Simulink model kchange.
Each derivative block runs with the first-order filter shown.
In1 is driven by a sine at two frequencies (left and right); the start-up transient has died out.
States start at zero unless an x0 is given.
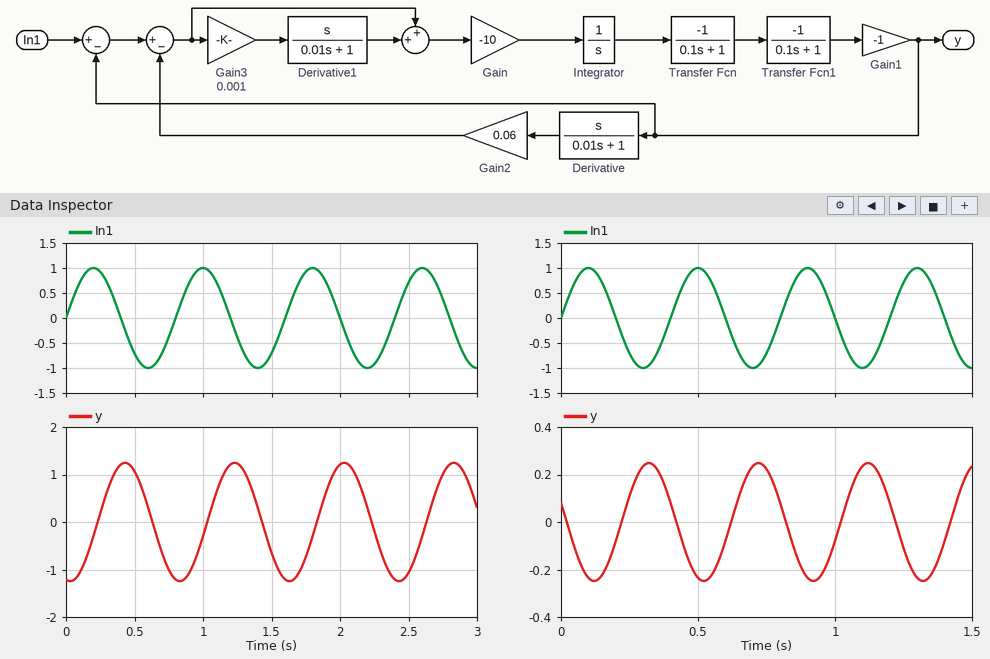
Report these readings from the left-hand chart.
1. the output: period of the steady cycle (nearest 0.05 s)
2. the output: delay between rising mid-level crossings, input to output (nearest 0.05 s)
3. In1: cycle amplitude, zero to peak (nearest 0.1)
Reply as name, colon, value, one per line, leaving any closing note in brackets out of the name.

the output: period of the steady cycle: 0.80 s
the output: delay between rising mid-level crossings, input to output: 0.25 s
In1: cycle amplitude, zero to peak: 1.0
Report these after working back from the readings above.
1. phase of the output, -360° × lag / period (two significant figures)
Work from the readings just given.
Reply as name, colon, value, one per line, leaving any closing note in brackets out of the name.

phase of the output, -360° × lag / period: -110°
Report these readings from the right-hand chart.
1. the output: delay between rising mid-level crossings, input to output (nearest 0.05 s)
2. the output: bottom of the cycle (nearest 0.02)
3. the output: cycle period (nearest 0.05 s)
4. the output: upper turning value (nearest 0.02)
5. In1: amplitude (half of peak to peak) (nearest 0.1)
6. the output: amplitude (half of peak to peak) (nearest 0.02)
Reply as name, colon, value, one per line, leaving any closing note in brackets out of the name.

the output: delay between rising mid-level crossings, input to output: 0.20 s
the output: bottom of the cycle: -0.24
the output: cycle period: 0.40 s
the output: upper turning value: 0.24
In1: amplitude (half of peak to peak): 1.0
the output: amplitude (half of peak to peak): 0.24
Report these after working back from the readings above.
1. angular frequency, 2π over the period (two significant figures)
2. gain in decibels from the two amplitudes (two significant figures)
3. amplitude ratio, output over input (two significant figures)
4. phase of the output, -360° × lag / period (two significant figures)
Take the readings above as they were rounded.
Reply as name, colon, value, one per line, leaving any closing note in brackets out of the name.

angular frequency, 2π over the period: 16 rad/s
gain in decibels from the two amplitudes: -12 dB
amplitude ratio, output over input: 0.24
phase of the output, -360° × lag / period: -180°
